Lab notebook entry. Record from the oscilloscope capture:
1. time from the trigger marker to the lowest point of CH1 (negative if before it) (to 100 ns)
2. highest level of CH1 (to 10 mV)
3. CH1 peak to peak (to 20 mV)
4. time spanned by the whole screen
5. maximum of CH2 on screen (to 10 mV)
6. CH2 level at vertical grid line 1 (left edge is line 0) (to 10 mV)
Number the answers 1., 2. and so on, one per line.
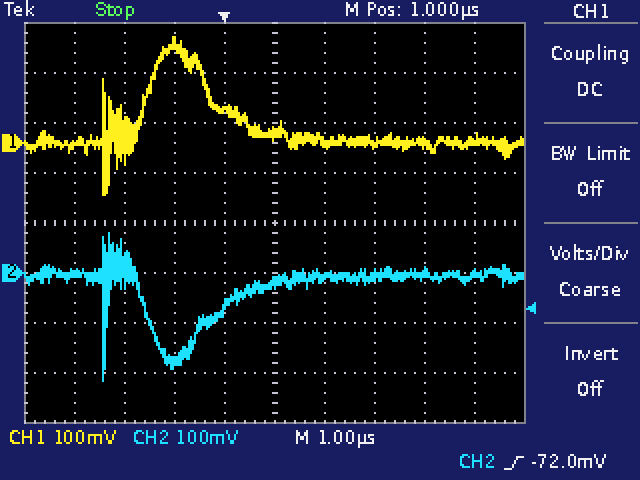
1. -2.4 µs
2. 210 mV
3. 320 mV
4. 10 µs
5. 80 mV
6. 0 mV
